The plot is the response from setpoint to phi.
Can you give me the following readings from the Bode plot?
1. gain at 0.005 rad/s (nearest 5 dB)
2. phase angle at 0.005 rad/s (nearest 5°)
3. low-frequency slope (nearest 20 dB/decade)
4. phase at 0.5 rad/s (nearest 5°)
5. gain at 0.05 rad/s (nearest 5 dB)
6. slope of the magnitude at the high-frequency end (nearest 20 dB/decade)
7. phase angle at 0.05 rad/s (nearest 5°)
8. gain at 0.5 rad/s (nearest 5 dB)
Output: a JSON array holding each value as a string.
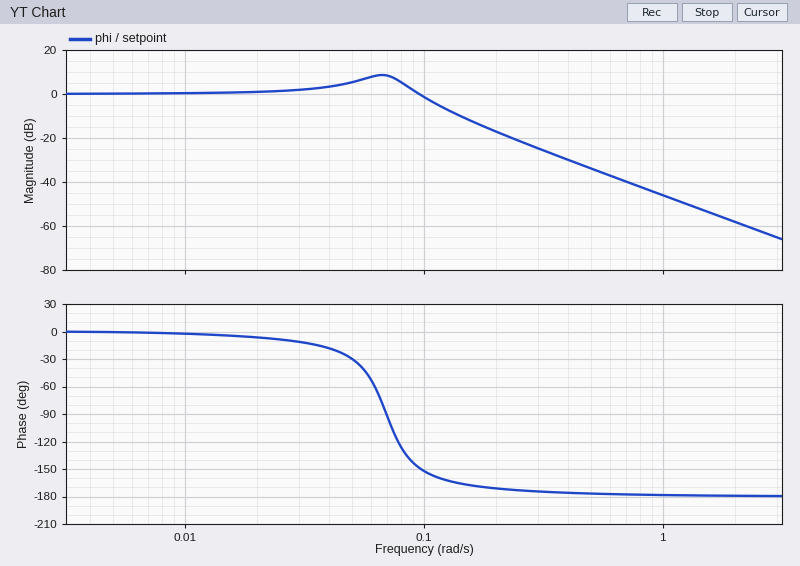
["0 dB", "0°", "0 dB/decade", "-175°", "5 dB", "-40 dB/decade", "-30°", "-35 dB"]
